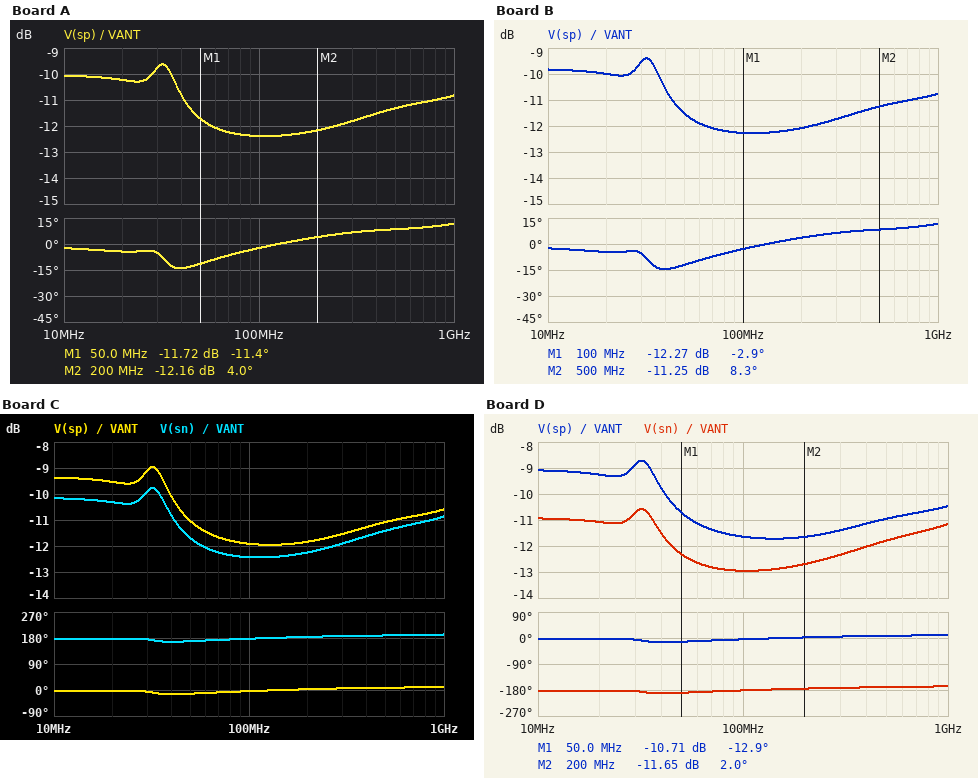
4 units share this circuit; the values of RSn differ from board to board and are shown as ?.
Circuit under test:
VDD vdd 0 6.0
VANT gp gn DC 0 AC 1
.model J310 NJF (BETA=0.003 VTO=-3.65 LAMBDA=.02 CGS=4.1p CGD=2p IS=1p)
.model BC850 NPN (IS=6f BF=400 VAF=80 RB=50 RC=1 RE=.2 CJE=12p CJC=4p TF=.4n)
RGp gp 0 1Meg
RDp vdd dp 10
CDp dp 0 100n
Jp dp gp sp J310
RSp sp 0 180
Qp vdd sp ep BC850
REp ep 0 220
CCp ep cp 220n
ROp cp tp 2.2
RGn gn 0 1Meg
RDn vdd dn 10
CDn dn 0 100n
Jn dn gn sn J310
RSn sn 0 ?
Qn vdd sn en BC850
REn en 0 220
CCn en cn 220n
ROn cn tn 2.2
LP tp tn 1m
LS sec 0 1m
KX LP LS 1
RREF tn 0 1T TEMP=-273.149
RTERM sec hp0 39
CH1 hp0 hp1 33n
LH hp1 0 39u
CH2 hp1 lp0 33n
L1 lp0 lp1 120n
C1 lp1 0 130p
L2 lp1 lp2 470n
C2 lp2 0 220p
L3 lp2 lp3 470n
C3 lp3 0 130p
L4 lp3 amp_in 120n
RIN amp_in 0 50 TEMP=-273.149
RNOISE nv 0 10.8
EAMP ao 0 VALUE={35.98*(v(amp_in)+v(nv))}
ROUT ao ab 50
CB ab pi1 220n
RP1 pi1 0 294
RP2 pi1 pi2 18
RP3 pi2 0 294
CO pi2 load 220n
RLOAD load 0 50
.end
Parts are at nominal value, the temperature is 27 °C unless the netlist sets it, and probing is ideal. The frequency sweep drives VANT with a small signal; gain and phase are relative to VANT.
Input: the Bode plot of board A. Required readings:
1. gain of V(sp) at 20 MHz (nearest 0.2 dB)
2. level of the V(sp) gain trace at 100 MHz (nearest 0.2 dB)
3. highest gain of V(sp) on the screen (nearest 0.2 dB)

-10.2 dB
-12.4 dB
-9.6 dB
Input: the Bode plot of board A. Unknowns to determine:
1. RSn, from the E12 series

270 Ω
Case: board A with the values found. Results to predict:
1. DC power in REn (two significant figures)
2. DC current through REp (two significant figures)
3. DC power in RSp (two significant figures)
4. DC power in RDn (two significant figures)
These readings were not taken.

8.7 mW
5.2 mA
19 mW
610 µW
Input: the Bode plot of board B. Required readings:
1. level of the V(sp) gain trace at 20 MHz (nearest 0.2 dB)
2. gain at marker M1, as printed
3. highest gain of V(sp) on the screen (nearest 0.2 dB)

-10.0 dB
-12.27 dB
-9.4 dB
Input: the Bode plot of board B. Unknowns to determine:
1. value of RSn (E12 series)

220 Ω
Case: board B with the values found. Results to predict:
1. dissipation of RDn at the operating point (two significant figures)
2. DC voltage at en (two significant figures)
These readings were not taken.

810 µW
1.3 V
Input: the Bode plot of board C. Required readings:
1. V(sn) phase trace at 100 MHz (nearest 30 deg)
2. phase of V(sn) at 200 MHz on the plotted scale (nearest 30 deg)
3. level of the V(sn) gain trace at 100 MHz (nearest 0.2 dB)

180 deg
180 deg
-12.4 dB
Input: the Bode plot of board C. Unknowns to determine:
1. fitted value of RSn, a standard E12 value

150 Ω
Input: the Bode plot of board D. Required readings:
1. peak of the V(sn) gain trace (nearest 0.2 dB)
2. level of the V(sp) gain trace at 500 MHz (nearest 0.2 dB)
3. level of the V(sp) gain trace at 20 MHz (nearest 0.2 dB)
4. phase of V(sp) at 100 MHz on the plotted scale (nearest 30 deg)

-10.6 dB
-11.0 dB
-9.2 dB
0 deg
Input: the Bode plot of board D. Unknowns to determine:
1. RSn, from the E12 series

120 Ω
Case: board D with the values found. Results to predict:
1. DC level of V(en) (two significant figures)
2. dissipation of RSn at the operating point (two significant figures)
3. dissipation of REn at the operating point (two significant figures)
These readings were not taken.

910 mV
22 mW
3.8 mW
